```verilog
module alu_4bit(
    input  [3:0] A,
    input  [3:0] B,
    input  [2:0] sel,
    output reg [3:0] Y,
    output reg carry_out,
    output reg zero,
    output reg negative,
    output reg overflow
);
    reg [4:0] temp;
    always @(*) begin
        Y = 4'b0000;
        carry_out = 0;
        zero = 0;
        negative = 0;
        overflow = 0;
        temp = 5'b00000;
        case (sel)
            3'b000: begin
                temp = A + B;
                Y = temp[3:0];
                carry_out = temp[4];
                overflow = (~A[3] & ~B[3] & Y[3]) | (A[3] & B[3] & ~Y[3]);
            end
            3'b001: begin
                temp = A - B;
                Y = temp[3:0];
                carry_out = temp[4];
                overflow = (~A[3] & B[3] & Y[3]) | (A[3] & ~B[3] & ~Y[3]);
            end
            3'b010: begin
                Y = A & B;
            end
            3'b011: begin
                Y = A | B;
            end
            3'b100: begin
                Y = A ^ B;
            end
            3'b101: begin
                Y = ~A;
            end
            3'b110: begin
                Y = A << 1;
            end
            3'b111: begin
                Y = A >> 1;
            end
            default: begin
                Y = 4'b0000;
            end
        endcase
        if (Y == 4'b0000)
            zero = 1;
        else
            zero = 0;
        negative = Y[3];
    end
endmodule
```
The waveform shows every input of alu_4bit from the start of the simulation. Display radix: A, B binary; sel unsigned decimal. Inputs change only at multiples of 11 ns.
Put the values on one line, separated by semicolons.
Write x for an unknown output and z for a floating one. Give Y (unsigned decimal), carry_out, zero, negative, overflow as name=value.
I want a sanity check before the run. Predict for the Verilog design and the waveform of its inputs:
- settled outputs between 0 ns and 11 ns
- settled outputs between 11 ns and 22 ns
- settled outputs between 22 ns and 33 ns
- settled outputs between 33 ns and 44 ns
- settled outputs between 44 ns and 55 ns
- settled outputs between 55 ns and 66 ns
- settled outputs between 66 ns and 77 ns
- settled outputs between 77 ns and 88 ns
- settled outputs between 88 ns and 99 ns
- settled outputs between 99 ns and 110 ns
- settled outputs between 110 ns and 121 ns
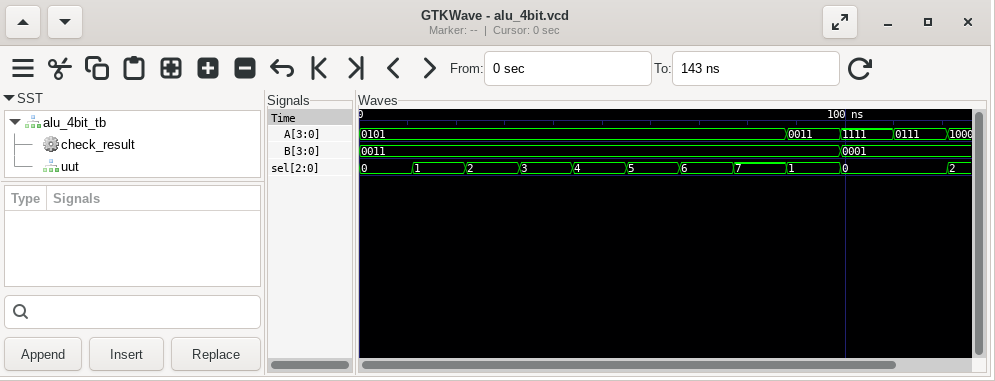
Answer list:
Y=8, carry_out=0, zero=0, negative=1, overflow=1; Y=2, carry_out=0, zero=0, negative=0, overflow=0; Y=1, carry_out=0, zero=0, negative=0, overflow=0; Y=7, carry_out=0, zero=0, negative=0, overflow=0; Y=6, carry_out=0, zero=0, negative=0, overflow=0; Y=10, carry_out=0, zero=0, negative=1, overflow=0; Y=10, carry_out=0, zero=0, negative=1, overflow=0; Y=2, carry_out=0, zero=0, negative=0, overflow=0; Y=0, carry_out=0, zero=1, negative=0, overflow=0; Y=0, carry_out=1, zero=1, negative=0, overflow=0; Y=8, carry_out=0, zero=0, negative=1, overflow=1
